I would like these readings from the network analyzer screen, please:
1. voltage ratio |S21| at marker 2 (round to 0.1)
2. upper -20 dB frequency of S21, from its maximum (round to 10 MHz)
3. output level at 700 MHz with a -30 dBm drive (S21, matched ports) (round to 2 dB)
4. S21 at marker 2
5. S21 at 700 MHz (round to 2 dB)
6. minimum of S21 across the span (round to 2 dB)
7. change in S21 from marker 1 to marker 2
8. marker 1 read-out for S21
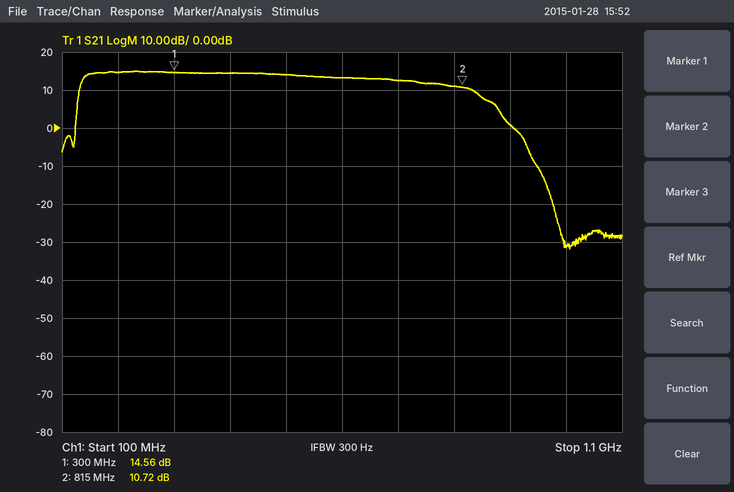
3.4
930 MHz
-18 dBm
10.72 dB
12 dB
-32 dB
-3.84 dB
14.56 dB
